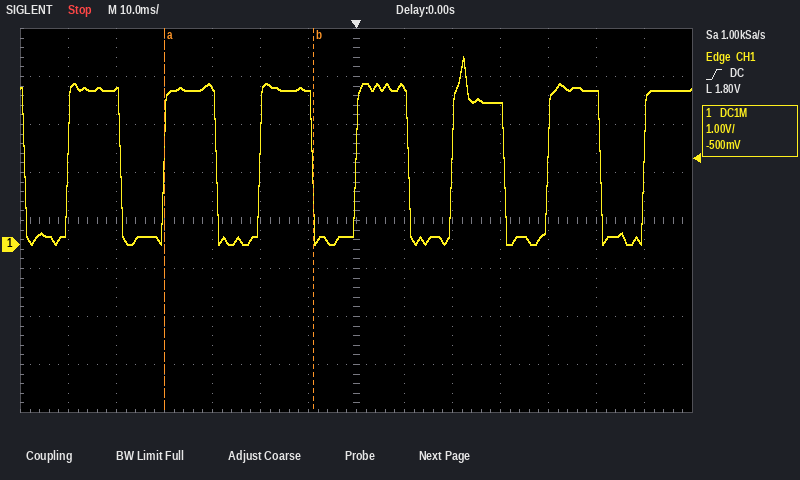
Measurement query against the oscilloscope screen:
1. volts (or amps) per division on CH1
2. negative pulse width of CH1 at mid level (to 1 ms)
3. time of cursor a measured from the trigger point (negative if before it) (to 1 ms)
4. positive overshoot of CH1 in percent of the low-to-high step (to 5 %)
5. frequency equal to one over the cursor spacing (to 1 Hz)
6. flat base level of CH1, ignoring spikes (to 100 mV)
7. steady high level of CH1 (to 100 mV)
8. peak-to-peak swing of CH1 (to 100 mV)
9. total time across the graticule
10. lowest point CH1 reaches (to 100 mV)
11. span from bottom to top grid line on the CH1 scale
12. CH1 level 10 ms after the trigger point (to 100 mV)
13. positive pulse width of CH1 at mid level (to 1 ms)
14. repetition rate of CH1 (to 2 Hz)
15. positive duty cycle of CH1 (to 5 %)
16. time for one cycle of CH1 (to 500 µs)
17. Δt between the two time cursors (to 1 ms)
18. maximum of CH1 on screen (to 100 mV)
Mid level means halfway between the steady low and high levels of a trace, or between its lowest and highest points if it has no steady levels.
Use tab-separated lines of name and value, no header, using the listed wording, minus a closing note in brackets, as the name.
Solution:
volts (or amps) per division on CH1	1 V
negative pulse width of CH1 at mid level	9 ms
time of cursor a measured from the trigger point (negative if before it)	-40 ms
positive overshoot of CH1 in percent of the low-to-high step	25 %
frequency equal to one over the cursor spacing	32 Hz
flat base level of CH1, ignoring spikes	200 mV
steady high level of CH1	3.2 V
peak-to-peak swing of CH1	3.9 V
total time across the graticule	140 ms
lowest point CH1 reaches	0.0 V
span from bottom to top grid line on the CH1 scale	8 V
CH1 level 10 ms after the trigger point	3.3 V
positive pulse width of CH1 at mid level	11 ms
repetition rate of CH1	50 Hz
positive duty cycle of CH1	55 %
time for one cycle of CH1	20.0 ms
Δt between the two time cursors	31 ms
maximum of CH1 on screen	3.9 V
